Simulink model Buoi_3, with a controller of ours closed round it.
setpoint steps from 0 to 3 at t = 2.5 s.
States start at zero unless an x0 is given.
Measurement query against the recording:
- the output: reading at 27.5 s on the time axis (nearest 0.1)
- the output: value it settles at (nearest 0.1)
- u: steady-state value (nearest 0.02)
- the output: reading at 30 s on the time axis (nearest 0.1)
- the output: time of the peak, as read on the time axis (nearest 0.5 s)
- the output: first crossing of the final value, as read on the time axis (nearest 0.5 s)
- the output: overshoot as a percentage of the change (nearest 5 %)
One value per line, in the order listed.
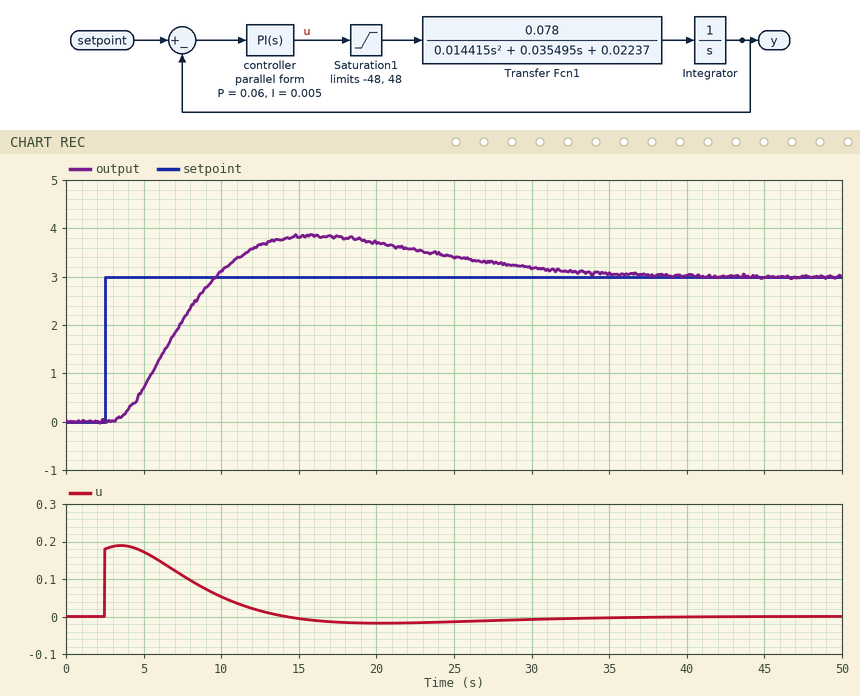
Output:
3.3
3.0
0.00
3.2
16.0 s
9.5 s
30 %
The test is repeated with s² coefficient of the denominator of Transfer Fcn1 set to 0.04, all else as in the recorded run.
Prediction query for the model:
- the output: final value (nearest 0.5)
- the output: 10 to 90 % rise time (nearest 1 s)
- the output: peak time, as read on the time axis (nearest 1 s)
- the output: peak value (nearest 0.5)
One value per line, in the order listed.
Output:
3.0
4 s
14 s
4.0
